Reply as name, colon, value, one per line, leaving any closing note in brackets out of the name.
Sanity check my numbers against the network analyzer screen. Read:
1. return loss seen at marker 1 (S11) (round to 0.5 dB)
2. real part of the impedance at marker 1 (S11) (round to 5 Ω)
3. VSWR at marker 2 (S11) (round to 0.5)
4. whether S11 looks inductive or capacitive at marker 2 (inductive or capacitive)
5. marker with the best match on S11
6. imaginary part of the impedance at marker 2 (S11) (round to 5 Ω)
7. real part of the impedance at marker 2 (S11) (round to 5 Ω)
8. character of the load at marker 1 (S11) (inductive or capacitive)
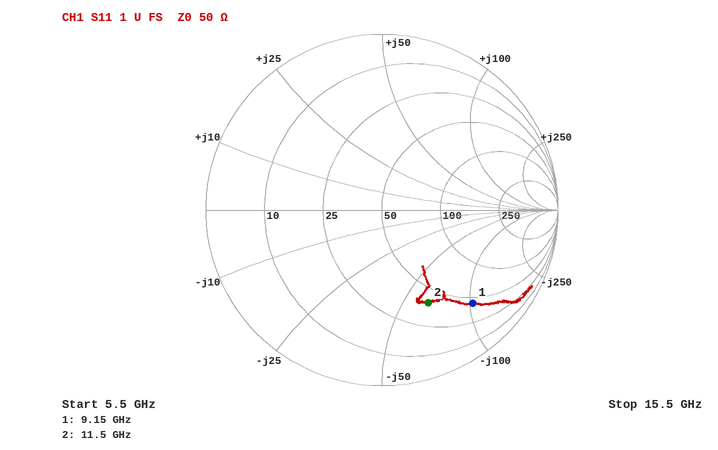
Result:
return loss seen at marker 1 (S11): 2.5 dB
real part of the impedance at marker 1 (S11): 45 Ω
VSWR at marker 2 (S11): 4.0
whether S11 looks inductive or capacitive at marker 2: capacitive
marker with the best match on S11: marker 2
imaginary part of the impedance at marker 2 (S11): -65 Ω
real part of the impedance at marker 2 (S11): 40 Ω
character of the load at marker 1 (S11): capacitive
